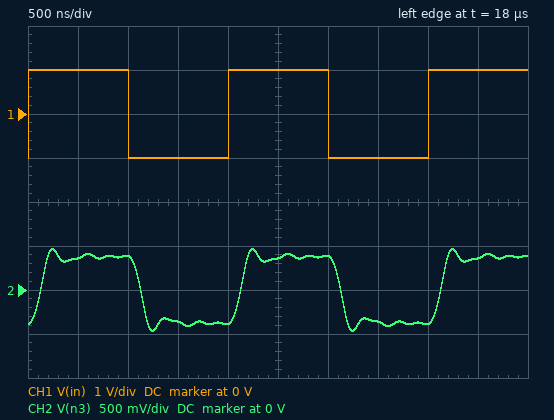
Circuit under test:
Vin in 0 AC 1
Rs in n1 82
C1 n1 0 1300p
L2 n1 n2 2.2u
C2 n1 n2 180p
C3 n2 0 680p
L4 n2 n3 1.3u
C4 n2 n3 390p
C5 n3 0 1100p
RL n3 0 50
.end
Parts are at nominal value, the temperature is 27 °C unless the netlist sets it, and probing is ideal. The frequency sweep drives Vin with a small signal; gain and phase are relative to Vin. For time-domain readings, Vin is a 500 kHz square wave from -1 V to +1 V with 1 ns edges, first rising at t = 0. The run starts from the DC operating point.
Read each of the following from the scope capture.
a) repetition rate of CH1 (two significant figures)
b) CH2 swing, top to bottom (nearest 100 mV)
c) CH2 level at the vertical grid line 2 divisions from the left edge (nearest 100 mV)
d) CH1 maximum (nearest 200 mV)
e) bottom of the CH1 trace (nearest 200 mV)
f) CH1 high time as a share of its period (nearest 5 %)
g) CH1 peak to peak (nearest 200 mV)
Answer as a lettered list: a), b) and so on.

a) 500 kHz
b) 900 mV
c) 400 mV
d) 1.0 V
e) -1.0 V
f) 50 %
g) 2.0 V
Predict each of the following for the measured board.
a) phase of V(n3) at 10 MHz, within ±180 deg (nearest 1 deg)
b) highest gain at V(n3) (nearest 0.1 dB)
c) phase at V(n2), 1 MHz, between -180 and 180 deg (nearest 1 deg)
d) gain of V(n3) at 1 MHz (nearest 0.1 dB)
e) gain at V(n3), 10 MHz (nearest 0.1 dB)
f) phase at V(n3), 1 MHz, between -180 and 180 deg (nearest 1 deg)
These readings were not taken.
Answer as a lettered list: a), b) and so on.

a) -68 deg
b) -8.2 dB
c) -32 deg
d) -8.9 dB
e) -56.7 dB
f) -42 deg
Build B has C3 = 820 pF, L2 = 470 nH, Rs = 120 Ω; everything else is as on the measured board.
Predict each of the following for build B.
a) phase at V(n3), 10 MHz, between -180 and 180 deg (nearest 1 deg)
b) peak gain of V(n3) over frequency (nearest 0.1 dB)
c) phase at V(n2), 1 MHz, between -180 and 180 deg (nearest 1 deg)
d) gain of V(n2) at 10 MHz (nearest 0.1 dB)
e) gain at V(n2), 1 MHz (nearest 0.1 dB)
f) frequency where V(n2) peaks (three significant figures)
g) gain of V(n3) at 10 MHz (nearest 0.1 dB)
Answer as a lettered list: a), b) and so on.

a) 115 deg
b) -10.6 dB
c) -30 deg
d) -19.9 dB
e) -12.2 dB
f) 8.61 MHz
g) -36.6 dB
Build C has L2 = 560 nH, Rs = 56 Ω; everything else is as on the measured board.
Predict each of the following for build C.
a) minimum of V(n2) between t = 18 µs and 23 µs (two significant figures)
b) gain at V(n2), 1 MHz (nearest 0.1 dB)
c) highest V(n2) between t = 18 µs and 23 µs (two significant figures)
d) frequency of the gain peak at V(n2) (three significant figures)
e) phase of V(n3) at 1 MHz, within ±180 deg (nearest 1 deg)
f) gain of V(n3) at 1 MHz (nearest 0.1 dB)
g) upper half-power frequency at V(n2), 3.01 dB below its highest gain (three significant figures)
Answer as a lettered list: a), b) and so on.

a) -590 mV
b) -7.5 dB
c) 590 mV
d) 8.17 MHz
e) -34 deg
f) -7.1 dB
g) 8.41 MHz
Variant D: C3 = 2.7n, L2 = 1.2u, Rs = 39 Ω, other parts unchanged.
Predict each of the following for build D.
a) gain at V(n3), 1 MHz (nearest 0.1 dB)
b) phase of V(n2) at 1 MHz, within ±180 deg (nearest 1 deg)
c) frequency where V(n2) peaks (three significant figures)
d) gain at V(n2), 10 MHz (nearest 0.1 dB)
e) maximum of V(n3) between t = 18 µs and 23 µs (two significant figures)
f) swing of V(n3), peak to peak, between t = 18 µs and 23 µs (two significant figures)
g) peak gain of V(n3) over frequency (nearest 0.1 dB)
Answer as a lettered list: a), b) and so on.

a) -5.9 dB
b) -37 deg
c) 4.40 MHz
d) -49.5 dB
e) 660 mV
f) 1.3 V
g) -5.0 dB
